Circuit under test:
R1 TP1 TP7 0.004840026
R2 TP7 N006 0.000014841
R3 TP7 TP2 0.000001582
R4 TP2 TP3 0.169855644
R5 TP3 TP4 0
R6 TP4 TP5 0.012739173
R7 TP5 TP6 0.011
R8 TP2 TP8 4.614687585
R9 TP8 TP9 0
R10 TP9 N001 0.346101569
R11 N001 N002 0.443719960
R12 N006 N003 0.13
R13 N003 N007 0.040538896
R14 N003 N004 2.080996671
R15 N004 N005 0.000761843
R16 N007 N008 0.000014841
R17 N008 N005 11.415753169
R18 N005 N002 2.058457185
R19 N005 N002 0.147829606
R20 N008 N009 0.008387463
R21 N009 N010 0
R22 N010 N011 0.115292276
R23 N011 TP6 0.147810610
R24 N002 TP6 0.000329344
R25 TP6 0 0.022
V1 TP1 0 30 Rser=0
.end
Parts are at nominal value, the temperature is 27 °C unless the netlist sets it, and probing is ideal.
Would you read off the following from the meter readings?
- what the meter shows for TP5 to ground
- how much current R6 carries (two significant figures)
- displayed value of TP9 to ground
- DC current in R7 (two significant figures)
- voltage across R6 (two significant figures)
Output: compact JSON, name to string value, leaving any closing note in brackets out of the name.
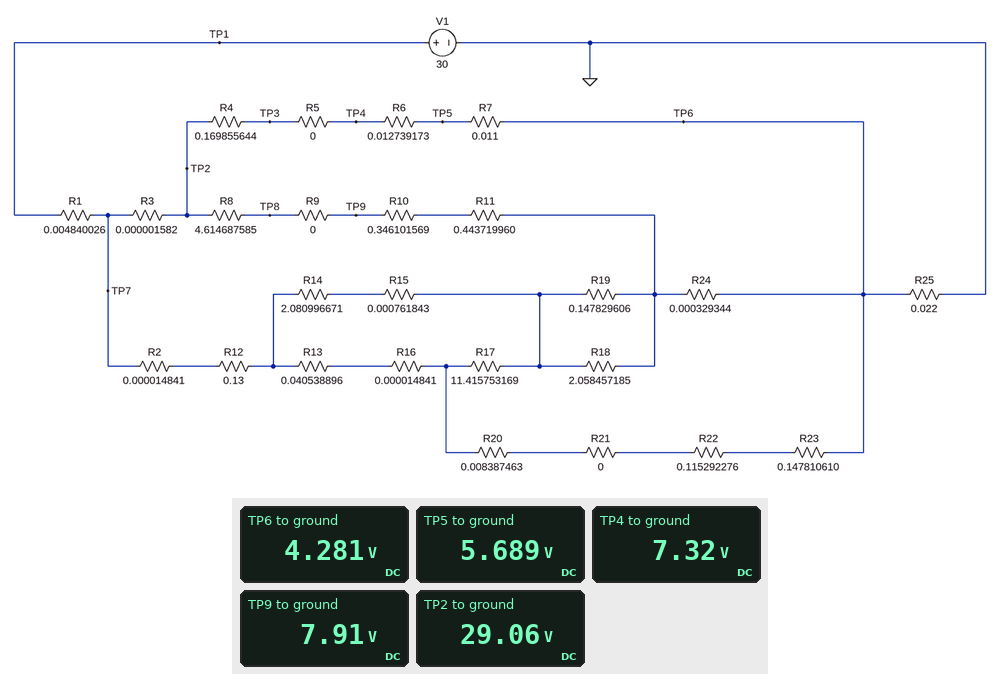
{"what the meter shows for TP5 to ground": "5.689 V", "how much current R6 carries": "130 A", "displayed value of TP9 to ground": "7.91 V", "DC current in R7": "130 A", "voltage across R6": "1.6 V"}
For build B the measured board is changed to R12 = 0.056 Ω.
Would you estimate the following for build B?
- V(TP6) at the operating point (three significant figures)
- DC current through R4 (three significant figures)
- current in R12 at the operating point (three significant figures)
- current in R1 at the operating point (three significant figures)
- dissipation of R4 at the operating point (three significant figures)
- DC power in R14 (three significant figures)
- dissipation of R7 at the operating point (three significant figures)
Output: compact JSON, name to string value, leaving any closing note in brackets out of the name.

{"V(TP6) at the operating point": "4.53 V", "DC current through R4": "126 A", "current in R12 at the operating point": "75.2 A", "current in R1 at the operating point": "206 A", "dissipation of R4 at the operating point": "2.71 kW", "DC power in R14": "170 W", "dissipation of R7 at the operating point": "176 W"}
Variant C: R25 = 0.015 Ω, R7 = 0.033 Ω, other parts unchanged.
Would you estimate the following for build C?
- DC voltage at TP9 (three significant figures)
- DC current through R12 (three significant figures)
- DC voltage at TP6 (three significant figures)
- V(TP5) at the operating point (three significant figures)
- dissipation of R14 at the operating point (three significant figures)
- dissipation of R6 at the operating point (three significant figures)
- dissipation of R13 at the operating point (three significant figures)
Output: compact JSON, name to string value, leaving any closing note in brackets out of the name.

{"DC voltage at TP9": "6.71 V", "DC current through R12": "65.6 A", "DC voltage at TP6": "2.88 V", "V(TP5) at the operating point": "6.89 V", "dissipation of R14 at the operating point": "129 W", "dissipation of R6 at the operating point": "188 W", "dissipation of R13 at the operating point": "135 W"}
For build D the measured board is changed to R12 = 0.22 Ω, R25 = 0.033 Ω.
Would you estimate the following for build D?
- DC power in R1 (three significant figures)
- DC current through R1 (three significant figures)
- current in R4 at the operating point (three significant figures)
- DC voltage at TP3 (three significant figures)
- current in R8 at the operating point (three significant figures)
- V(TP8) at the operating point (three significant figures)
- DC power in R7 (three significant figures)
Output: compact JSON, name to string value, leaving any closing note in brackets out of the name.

{"DC power in R1": "145 W", "DC current through R1": "173 A", "current in R4 at the operating point": "121 A", "DC voltage at TP3": "8.59 V", "current in R8 at the operating point": "4.34 A", "V(TP8) at the operating point": "9.15 V", "DC power in R7": "161 W"}
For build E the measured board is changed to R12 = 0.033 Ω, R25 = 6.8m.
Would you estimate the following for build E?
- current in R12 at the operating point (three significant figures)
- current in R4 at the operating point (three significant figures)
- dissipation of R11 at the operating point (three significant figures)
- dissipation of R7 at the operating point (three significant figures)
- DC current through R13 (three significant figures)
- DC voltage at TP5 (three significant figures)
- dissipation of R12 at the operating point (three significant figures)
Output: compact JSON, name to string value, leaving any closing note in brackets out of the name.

{"current in R12 at the operating point": "90.1 A", "current in R4 at the operating point": "141 A", "dissipation of R11 at the operating point": "11.3 W", "dissipation of R7 at the operating point": "218 W", "DC current through R13": "79.3 A", "DC voltage at TP5": "3.15 V", "dissipation of R12 at the operating point": "268 W"}
